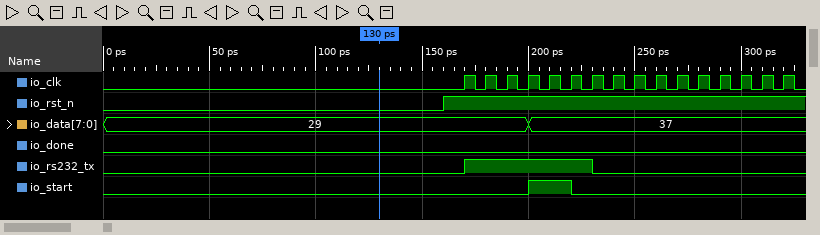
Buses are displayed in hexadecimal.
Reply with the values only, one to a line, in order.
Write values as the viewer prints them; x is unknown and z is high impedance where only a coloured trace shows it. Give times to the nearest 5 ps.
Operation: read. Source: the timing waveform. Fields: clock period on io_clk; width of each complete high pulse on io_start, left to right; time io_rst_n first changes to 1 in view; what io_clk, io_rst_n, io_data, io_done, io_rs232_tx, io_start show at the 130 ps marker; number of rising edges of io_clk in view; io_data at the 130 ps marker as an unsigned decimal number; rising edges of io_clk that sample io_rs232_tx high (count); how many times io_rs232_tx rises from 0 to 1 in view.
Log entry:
10 ps
20 ps
160 ps
io_clk=0, io_rst_n=0, io_data=29, io_done=0, io_rs232_tx=0, io_start=0
16
41
6
1
